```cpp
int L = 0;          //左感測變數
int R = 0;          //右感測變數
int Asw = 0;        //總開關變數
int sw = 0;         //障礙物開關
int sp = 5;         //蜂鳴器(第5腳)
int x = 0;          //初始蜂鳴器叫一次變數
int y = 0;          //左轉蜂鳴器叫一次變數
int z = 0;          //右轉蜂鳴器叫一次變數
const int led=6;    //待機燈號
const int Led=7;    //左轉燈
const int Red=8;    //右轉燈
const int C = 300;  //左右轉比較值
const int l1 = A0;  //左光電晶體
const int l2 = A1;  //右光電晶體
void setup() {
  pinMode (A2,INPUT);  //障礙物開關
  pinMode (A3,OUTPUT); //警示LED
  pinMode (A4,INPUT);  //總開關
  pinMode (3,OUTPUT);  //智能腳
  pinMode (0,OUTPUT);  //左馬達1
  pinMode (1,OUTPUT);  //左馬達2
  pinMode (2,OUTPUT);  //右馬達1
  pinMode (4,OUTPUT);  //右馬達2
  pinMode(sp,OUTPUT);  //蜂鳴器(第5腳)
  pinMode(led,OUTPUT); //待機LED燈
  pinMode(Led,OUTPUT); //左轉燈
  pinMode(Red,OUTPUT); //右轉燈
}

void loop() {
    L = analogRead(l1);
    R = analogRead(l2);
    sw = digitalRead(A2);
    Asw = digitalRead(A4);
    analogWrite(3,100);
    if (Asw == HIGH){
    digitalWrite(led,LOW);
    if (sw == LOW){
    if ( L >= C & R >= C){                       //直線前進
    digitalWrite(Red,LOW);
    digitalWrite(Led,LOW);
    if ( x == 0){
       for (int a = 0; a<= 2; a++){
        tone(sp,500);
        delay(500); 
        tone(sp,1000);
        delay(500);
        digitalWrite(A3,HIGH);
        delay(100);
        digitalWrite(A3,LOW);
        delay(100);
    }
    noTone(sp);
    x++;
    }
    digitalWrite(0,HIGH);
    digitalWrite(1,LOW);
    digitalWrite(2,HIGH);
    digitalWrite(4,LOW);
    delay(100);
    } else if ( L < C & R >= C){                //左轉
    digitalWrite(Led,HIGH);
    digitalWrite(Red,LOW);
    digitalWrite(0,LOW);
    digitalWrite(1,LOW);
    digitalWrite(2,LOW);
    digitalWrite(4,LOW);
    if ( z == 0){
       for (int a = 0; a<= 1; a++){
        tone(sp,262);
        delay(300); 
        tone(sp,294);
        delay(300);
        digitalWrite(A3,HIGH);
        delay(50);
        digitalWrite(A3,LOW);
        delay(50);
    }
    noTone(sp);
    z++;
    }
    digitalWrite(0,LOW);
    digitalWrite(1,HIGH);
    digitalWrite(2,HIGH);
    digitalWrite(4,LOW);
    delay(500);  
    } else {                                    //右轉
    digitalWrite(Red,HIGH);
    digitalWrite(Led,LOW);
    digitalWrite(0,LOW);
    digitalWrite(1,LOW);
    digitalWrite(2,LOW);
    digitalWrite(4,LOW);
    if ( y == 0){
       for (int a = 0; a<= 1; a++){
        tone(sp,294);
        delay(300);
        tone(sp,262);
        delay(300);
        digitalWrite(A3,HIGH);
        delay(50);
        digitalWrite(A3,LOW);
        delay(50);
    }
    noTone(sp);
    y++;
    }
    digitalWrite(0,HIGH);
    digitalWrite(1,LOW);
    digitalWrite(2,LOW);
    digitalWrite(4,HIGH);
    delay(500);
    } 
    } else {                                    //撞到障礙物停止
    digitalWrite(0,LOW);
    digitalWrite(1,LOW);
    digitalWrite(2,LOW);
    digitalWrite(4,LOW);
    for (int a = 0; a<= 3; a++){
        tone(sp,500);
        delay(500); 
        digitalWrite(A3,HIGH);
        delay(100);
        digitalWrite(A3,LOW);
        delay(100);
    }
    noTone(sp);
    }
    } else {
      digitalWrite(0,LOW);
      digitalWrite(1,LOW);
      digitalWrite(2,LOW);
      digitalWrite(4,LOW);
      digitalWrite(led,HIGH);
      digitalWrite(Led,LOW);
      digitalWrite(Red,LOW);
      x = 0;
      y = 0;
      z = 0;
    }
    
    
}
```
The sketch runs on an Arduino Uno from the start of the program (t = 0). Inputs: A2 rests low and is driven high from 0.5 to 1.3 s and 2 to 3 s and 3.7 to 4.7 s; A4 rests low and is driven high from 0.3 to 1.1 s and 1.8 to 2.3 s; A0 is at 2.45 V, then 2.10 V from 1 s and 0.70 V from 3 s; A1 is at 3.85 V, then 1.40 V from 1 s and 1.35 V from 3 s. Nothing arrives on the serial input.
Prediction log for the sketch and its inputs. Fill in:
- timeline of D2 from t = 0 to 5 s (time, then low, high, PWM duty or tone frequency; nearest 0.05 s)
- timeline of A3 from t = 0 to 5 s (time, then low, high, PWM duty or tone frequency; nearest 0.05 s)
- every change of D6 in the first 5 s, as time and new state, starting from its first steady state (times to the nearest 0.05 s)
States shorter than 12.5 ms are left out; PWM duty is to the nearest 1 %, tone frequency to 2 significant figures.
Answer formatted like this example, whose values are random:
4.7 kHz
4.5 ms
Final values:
0 s low; 3.9 s high; 4 s low
0 s low; 1.3 s high; 1.4 s low; 2.5 s high; 2.6 s low; 3.7 s high; 3.8 s low
0 s high; 0.3 s low; 4 s high
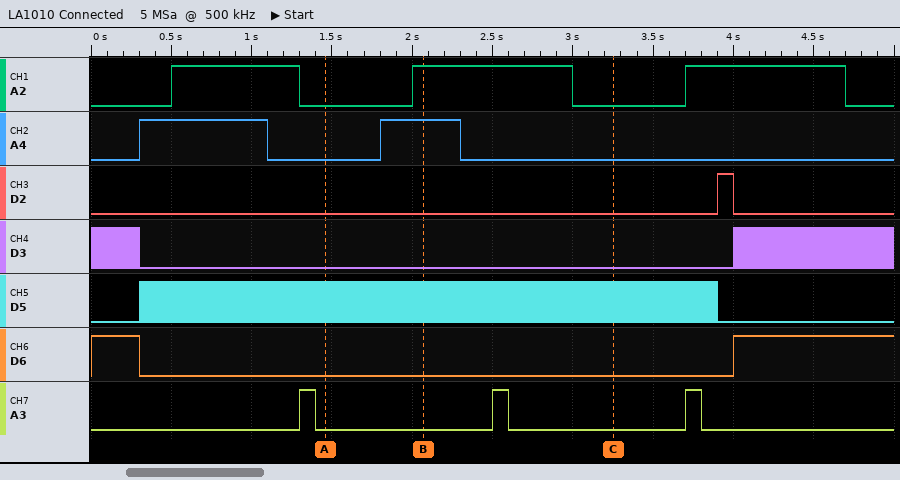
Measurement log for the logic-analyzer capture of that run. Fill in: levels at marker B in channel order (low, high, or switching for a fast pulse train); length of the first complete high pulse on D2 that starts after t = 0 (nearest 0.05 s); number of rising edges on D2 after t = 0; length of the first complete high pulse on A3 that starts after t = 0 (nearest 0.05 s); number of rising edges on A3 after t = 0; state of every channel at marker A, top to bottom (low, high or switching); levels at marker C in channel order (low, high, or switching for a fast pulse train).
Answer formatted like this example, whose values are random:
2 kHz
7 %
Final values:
A2 high, A4 high, D2 low, D3 low, D5 switching, D6 low, A3 low
0.10 s
1
0.10 s
3
A2 low, A4 low, D2 low, D3 low, D5 switching, D6 low, A3 low
A2 low, A4 low, D2 low, D3 low, D5 switching, D6 low, A3 low
